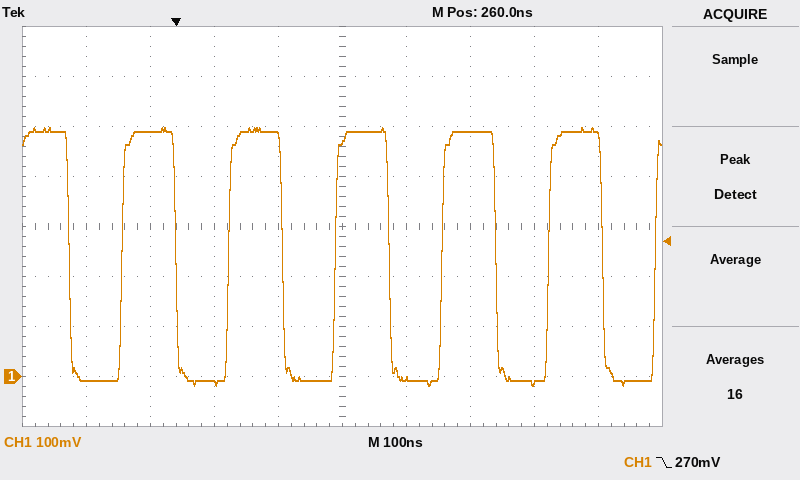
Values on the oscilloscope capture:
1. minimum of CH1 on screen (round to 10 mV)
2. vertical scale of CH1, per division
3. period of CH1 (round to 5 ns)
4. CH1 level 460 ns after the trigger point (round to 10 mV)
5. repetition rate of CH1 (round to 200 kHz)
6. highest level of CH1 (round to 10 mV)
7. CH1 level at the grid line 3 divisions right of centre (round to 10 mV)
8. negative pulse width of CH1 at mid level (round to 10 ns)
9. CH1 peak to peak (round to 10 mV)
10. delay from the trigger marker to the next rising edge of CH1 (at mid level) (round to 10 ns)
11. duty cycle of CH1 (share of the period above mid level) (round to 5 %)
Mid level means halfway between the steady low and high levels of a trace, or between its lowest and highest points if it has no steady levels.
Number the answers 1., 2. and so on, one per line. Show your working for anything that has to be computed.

1. -20 mV
2. 100 mV
3. 165 ns
4. 490 mV
5. 1 / 165 ns ≈ 6.06 MHz, so 6.0 MHz to the nearest 200 kHz
6. 500 mV
7. -10 mV
8. 80 ns
9. 500 mV − (-20 mV) = 520 mV
10. 80 ns
11. 50 %
